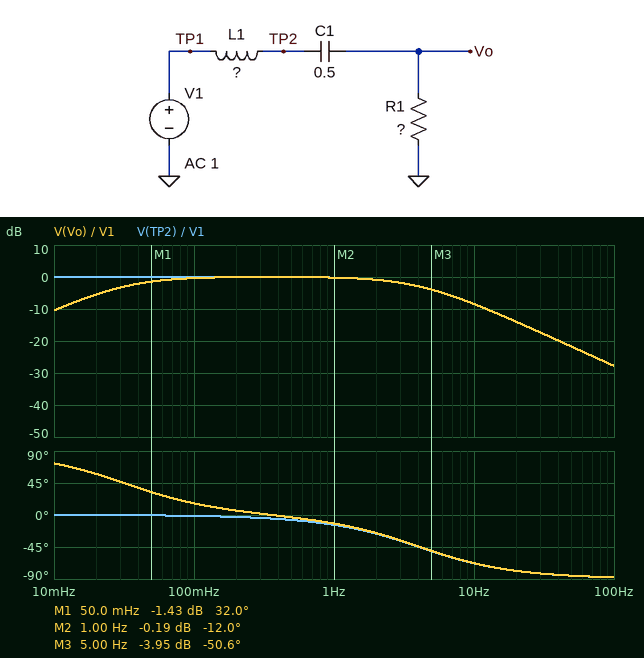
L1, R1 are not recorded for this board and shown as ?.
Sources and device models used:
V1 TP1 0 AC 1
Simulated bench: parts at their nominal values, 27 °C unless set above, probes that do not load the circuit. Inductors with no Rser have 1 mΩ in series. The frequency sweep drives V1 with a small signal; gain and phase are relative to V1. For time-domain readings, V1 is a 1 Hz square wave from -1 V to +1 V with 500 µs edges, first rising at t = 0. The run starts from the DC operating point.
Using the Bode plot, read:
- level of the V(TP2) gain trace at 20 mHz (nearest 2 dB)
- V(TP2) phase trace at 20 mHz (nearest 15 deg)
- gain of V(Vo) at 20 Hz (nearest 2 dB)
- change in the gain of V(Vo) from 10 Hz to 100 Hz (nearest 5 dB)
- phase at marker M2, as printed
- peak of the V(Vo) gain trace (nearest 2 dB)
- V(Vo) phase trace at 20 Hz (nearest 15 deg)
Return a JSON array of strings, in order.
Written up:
["0 dB", "0 deg", "-14 dB", "-20 dB", "-12.0 deg", "0 dB", "-75 deg"]
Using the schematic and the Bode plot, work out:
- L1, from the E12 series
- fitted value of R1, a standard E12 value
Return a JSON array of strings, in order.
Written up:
["390 mH", "10 Ω"]
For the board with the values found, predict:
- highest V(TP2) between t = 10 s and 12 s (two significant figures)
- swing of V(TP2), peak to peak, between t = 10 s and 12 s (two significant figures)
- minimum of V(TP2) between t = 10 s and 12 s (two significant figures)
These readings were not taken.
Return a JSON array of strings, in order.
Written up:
["1.0 V", "2.0 V", "-1.0 V"]
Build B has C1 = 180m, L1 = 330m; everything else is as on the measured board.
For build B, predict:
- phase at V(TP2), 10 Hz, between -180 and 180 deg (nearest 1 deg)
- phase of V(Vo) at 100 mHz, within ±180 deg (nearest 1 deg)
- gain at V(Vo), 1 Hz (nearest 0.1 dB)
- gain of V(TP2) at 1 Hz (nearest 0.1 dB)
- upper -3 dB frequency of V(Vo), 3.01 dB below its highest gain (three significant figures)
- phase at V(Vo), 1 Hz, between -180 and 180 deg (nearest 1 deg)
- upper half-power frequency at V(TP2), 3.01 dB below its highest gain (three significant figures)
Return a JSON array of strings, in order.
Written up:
["-65 deg", "41 deg", "-0.1 dB", "0 dB", "4.91 Hz", "-7 deg", "4.77 Hz"]
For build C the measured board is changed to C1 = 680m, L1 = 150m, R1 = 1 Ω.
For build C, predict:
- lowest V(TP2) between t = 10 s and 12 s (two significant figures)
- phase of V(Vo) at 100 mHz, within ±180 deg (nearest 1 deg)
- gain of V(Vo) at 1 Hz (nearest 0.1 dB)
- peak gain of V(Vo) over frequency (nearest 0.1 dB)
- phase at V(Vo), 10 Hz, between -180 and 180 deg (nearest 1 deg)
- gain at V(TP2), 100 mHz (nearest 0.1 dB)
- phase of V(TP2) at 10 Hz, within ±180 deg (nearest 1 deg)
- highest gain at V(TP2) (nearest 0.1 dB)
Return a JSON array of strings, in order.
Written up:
["-1.1 V", "66 deg", "-1.8 dB", "0 dB", "-84 deg", "0.3 dB", "-85 deg", "1.1 dB"]
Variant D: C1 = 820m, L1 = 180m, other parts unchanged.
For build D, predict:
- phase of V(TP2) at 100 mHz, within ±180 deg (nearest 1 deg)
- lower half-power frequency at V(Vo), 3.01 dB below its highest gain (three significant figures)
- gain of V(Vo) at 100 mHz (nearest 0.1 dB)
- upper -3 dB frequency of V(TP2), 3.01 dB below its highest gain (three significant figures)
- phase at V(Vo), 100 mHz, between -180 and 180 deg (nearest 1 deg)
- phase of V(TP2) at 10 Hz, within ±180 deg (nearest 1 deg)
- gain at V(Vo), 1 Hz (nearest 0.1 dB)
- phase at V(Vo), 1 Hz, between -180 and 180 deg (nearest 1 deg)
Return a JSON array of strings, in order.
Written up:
["-1 deg", "19.4 mHz", "-0.1 dB", "8.83 Hz", "10 deg", "-49 deg", "0 dB", "-5 deg"]
